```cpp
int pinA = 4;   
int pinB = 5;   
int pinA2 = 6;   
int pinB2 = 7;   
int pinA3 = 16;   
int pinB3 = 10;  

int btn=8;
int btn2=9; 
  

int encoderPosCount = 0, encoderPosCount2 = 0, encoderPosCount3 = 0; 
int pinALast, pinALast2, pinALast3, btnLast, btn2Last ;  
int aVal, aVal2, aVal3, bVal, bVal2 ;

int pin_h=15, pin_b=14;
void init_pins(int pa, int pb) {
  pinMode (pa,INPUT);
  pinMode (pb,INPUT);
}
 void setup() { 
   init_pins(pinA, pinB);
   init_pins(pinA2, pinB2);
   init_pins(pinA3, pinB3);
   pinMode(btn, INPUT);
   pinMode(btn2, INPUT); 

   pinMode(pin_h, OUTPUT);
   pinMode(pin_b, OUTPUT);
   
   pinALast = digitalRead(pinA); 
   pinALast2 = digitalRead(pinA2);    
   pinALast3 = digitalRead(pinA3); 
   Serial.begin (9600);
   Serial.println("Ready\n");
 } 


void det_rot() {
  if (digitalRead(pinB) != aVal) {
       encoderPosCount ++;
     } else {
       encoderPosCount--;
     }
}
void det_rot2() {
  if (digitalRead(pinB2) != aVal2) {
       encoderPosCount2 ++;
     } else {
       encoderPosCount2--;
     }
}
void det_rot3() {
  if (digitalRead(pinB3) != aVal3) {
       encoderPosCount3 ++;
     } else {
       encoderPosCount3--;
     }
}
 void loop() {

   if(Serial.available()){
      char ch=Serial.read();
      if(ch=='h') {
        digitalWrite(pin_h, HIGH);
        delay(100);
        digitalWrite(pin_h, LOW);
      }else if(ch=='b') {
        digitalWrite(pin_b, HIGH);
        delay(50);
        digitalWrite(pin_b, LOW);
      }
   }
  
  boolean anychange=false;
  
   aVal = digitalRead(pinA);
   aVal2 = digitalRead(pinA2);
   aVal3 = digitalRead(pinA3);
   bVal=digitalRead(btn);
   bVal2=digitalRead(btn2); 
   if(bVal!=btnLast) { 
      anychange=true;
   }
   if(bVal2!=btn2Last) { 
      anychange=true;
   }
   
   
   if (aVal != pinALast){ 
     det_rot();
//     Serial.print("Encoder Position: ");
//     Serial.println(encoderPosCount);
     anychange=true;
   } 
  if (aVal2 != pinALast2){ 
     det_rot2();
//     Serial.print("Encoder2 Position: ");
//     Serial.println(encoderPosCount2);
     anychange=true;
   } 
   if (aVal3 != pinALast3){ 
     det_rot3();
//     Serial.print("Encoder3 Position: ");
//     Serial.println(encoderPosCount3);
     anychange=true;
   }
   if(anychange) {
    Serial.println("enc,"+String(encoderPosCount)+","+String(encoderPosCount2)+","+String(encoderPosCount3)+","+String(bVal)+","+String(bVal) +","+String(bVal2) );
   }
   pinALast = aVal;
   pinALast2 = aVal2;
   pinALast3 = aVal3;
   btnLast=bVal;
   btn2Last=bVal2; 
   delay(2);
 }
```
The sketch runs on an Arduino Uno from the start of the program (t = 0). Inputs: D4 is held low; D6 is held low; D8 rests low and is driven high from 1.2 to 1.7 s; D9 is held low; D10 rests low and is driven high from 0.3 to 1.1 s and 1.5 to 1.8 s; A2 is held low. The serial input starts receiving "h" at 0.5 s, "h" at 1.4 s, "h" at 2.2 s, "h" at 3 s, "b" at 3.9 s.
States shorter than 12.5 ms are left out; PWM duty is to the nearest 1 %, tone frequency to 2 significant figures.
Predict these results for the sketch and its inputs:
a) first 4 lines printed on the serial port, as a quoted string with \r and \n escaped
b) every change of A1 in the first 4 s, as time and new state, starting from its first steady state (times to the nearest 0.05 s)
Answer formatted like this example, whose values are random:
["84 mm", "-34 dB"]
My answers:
["\"Ready\\n\\r\\nenc,0,0,0,1,1,0\\r\\nenc,0,0,0,0,0,0\\r\\n\"", "0 s low; 0.5 s high; 0.6 s low; 1.4 s high; 1.5 s low; 2.2 s high; 2.3 s low; 3 s high; 3.1 s low"]
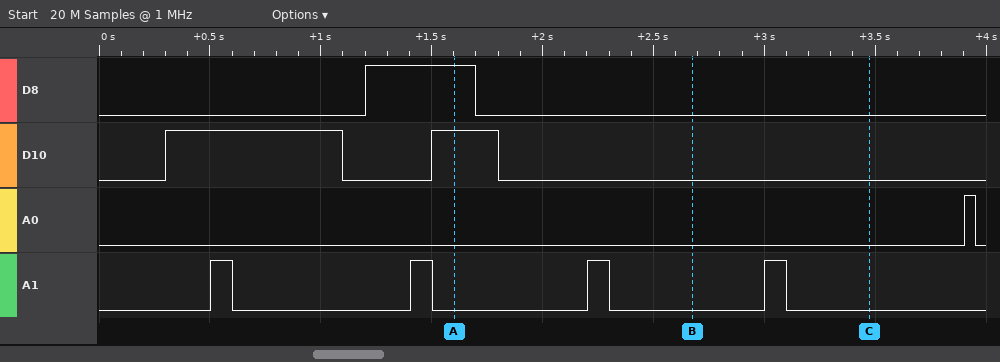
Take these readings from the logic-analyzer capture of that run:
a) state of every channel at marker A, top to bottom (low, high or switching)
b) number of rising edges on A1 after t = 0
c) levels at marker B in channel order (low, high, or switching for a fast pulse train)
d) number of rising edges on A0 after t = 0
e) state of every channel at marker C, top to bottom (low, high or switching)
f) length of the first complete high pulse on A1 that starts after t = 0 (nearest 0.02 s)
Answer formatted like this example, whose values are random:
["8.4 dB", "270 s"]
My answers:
["D8 high, D10 high, A0 low, A1 low", "4", "D8 low, D10 low, A0 low, A1 low", "1", "D8 low, D10 low, A0 low, A1 low", "0.10 s"]
